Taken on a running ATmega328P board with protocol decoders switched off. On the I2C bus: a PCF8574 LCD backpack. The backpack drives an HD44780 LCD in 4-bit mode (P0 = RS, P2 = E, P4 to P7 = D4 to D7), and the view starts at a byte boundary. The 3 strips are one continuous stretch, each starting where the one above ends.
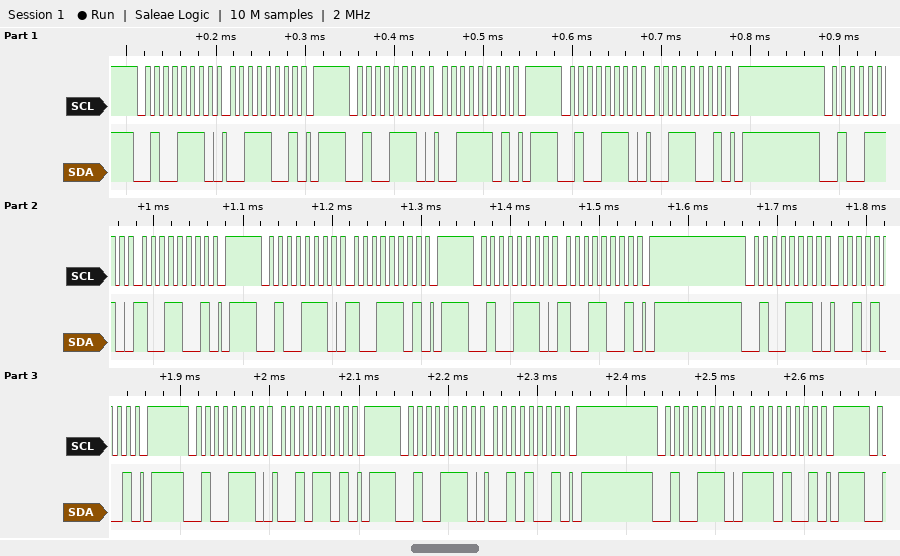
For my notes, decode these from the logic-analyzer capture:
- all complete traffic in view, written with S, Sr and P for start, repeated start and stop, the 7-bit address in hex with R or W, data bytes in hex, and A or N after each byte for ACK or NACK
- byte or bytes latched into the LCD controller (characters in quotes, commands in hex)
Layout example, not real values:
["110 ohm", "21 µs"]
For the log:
["S 27W A 39 A P S 27W A 3D A P S 27W A 39 A P S 27W A 99 A P S 27W A 9D A P S 27W A 99 A P S 27W A 29 A P S 27W A 2D A P S 27W A 29 A P S 27W A E9 A P", "'9'"]
